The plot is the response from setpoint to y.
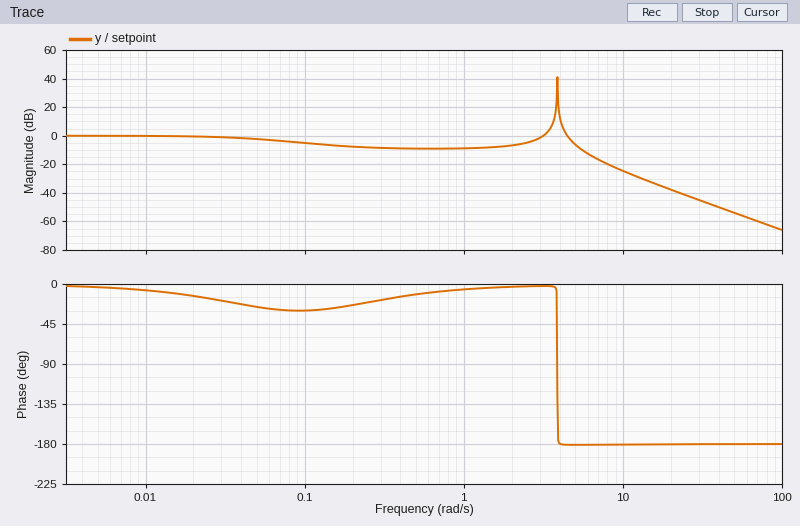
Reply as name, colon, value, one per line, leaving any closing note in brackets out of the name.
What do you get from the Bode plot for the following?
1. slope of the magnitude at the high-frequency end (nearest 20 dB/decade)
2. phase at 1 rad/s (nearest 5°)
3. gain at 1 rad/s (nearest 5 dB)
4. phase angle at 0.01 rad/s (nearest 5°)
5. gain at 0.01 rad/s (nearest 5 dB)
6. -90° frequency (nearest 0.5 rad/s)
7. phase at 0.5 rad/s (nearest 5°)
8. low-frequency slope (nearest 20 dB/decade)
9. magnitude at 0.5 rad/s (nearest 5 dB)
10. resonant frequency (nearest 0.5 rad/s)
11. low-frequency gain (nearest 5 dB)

slope of the magnitude at the high-frequency end: -40 dB/decade
phase at 1 rad/s: -5°
gain at 1 rad/s: -10 dB
phase angle at 0.01 rad/s: -5°
gain at 0.01 rad/s: 0 dB
-90° frequency: 4.0 rad/s
phase at 0.5 rad/s: -10°
low-frequency slope: 0 dB/decade
magnitude at 0.5 rad/s: -10 dB
resonant frequency: 4.0 rad/s
low-frequency gain: 0 dB
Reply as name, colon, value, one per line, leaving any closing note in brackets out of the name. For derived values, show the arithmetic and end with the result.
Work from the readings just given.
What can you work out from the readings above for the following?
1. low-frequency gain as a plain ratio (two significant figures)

low-frequency gain as a plain ratio: 10^(0 / 20) = 1.0
